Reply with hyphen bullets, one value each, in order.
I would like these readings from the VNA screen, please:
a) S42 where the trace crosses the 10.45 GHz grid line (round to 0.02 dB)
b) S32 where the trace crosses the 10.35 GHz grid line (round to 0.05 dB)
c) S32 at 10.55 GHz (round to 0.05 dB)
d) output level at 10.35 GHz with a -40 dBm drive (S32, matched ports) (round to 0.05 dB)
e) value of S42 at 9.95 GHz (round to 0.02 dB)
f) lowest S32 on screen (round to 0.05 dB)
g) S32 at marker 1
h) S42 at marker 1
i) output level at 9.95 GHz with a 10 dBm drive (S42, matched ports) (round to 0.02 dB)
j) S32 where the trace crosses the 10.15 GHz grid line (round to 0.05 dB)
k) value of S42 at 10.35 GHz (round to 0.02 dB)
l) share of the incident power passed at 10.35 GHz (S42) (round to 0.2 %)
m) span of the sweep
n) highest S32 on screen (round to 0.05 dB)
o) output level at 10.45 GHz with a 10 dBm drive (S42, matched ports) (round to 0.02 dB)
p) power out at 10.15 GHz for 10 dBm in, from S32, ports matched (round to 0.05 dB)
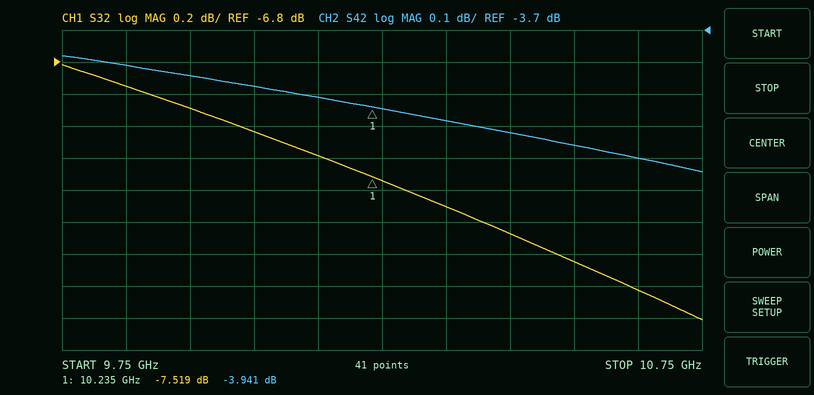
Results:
- -4.02 dB
- -7.70 dB
- -8.05 dB
- -47.70 dBm
- -3.84 dB
- -8.40 dB
- -7.519 dB
- -3.941 dB
- 6.16 dBm
- -7.40 dB
- -3.98 dB
- 40.0 %
- 1 GHz
- -6.80 dB
- 5.98 dBm
- 2.60 dBm
